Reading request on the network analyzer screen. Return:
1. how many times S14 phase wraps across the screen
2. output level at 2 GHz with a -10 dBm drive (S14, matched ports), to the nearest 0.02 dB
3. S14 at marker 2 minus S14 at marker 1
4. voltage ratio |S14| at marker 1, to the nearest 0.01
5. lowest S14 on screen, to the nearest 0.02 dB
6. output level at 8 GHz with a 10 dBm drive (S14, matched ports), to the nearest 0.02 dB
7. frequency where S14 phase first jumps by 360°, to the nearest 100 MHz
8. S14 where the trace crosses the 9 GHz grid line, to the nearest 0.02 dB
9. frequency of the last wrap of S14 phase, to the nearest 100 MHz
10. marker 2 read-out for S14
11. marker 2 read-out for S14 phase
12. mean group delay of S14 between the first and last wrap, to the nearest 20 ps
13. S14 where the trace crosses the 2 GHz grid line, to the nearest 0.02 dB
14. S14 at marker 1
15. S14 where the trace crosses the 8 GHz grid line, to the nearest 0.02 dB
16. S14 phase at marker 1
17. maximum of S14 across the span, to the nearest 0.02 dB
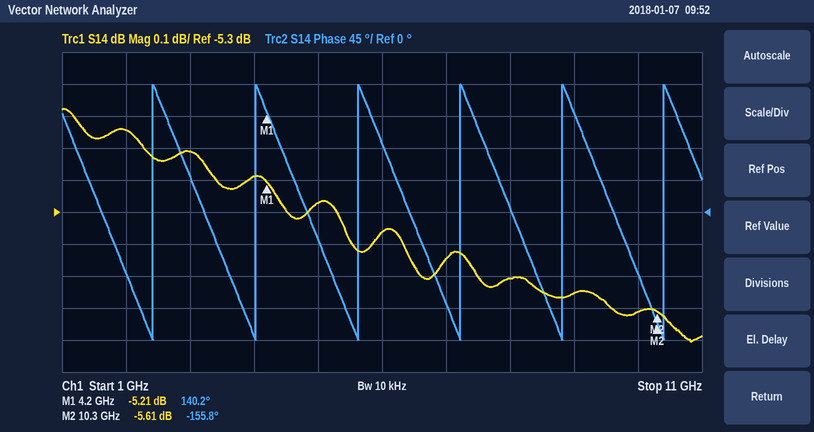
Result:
6
-15.04 dBm
-0.40 dB
0.55
-5.70 dB
4.50 dBm
2.4 GHz
-5.56 dB
10.4 GHz
-5.61 dB
-155.8°
620 ps
-5.04 dB
-5.21 dB
-5.50 dB
140.2°
-4.98 dB
